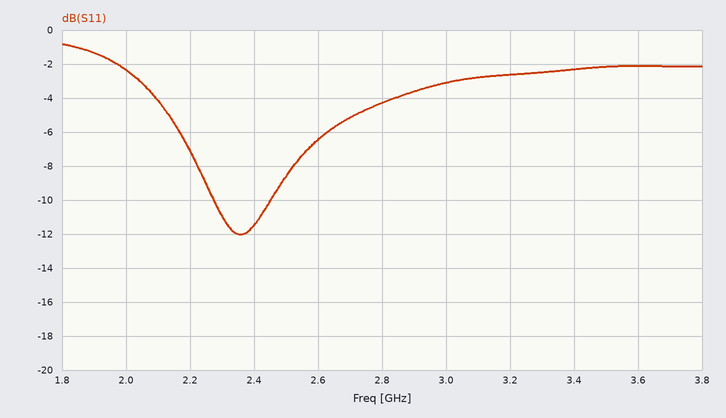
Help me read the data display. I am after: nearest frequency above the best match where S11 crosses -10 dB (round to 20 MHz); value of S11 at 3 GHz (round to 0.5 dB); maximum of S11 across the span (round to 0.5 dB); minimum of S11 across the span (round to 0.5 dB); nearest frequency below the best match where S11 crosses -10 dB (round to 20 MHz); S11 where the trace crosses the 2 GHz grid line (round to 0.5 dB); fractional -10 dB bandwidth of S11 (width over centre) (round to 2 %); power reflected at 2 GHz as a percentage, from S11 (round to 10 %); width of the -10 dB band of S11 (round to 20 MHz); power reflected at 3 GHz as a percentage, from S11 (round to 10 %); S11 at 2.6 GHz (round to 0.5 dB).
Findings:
2.46 GHz
-3.0 dB
-1.0 dB
-12.0 dB
2.28 GHz
-2.5 dB
8 %
60 %
180 MHz
50 %
-6.5 dB
